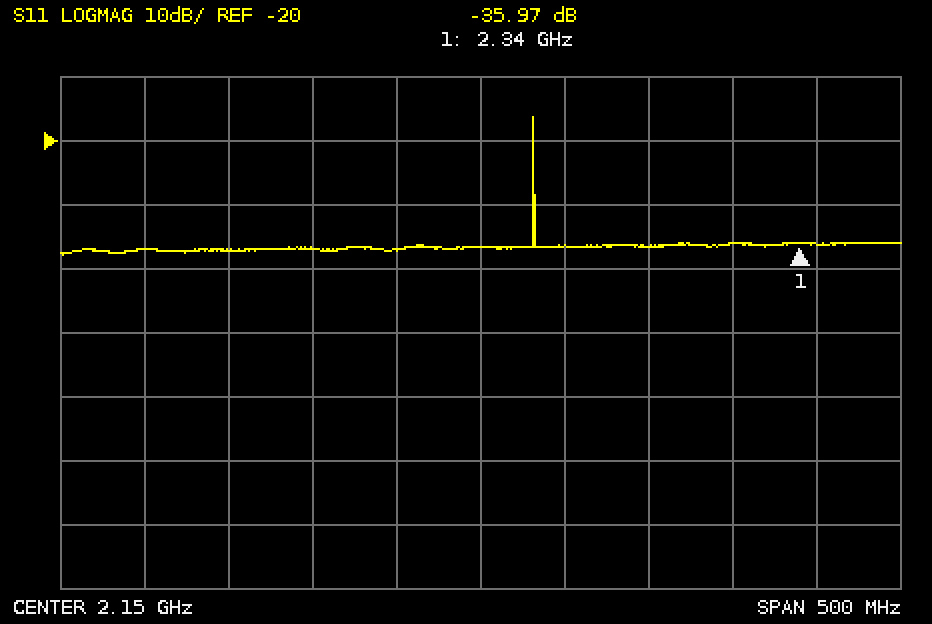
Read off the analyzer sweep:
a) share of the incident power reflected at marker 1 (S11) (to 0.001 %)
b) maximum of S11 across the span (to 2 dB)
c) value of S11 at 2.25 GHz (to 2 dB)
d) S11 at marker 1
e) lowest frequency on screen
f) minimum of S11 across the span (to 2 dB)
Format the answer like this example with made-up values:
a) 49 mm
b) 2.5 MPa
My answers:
a) 0.025 %
b) -16 dB
c) -36 dB
d) -35.97 dB
e) 1.9 GHz
f) -38 dB
